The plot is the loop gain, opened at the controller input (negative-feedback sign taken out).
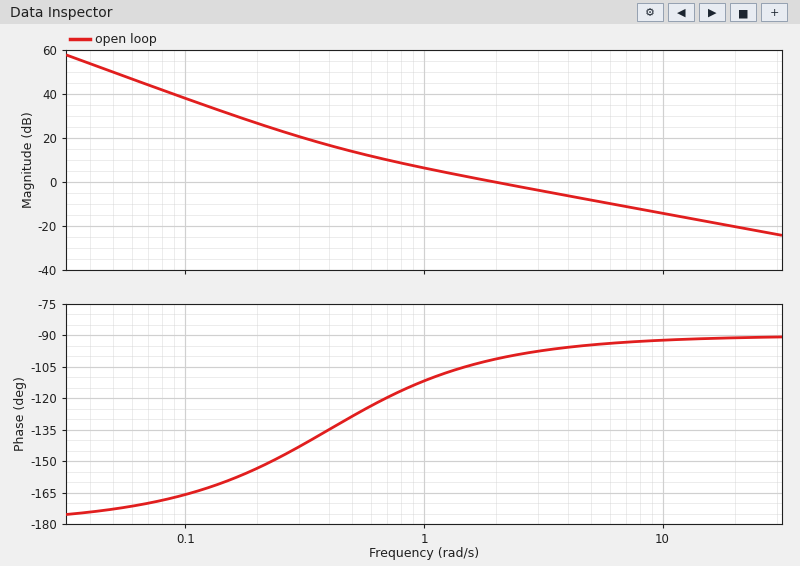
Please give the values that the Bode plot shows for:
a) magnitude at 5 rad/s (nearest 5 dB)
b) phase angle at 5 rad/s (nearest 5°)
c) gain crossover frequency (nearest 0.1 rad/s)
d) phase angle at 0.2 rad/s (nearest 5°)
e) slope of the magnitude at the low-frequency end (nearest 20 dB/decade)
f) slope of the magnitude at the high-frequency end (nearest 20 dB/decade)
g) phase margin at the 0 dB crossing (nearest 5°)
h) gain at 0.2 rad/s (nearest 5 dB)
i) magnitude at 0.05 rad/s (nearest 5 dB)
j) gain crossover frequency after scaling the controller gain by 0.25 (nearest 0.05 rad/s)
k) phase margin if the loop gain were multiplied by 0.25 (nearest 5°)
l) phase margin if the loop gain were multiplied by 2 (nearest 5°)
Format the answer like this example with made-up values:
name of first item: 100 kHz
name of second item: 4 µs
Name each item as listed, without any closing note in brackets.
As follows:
magnitude at 5 rad/s: -10 dB
phase angle at 5 rad/s: -95°
gain crossover frequency: 2.0 rad/s
phase angle at 0.2 rad/s: -155°
slope of the magnitude at the low-frequency end: -40 dB/decade
slope of the magnitude at the high-frequency end: -20 dB/decade
phase margin at the 0 dB crossing: 80°
gain at 0.2 rad/s: 25 dB
magnitude at 0.05 rad/s: 50 dB
gain crossover frequency after scaling the controller gain by 0.25: 0.60 rad/s
phase margin if the loop gain were multiplied by 0.25: 55°
phase margin if the loop gain were multiplied by 2: 85°
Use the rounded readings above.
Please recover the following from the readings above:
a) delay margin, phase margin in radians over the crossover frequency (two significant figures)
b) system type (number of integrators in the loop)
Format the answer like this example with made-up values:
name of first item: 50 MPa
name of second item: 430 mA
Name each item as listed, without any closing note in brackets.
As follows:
delay margin, phase margin in radians over the crossover frequency: 0.70 s
system type: 2
